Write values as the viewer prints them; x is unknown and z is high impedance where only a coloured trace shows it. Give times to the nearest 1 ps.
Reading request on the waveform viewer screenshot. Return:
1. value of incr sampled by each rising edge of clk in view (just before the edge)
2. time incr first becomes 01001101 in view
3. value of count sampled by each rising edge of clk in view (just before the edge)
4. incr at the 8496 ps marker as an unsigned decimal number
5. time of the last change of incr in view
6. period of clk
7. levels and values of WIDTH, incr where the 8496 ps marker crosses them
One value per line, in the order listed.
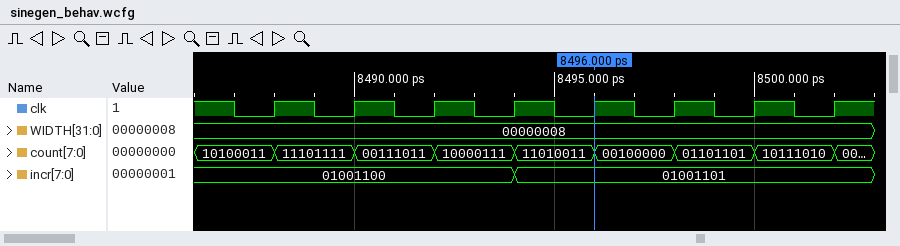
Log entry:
01001100, 01001100, 01001100, 01001100, 01001101, 01001101, 01001101, 01001101
8494 ps
10100011, 11101111, 00111011, 10000111, 11010011, 00100000, 01101101, 10111010
77
8494 ps
2 ps
WIDTH=00000008, incr=01001101
